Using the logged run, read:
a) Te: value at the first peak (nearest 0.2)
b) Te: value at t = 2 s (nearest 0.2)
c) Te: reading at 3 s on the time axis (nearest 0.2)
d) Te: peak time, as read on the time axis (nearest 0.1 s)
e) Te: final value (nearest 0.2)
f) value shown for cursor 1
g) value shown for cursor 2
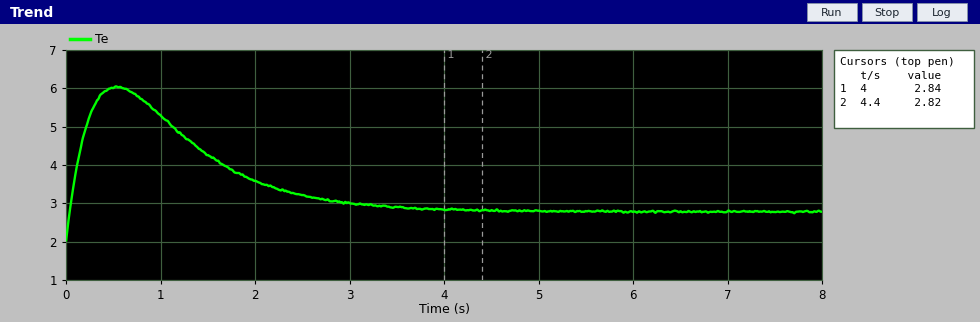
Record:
6.0
3.6
3.0
0.5 s
2.8
2.84
2.82
